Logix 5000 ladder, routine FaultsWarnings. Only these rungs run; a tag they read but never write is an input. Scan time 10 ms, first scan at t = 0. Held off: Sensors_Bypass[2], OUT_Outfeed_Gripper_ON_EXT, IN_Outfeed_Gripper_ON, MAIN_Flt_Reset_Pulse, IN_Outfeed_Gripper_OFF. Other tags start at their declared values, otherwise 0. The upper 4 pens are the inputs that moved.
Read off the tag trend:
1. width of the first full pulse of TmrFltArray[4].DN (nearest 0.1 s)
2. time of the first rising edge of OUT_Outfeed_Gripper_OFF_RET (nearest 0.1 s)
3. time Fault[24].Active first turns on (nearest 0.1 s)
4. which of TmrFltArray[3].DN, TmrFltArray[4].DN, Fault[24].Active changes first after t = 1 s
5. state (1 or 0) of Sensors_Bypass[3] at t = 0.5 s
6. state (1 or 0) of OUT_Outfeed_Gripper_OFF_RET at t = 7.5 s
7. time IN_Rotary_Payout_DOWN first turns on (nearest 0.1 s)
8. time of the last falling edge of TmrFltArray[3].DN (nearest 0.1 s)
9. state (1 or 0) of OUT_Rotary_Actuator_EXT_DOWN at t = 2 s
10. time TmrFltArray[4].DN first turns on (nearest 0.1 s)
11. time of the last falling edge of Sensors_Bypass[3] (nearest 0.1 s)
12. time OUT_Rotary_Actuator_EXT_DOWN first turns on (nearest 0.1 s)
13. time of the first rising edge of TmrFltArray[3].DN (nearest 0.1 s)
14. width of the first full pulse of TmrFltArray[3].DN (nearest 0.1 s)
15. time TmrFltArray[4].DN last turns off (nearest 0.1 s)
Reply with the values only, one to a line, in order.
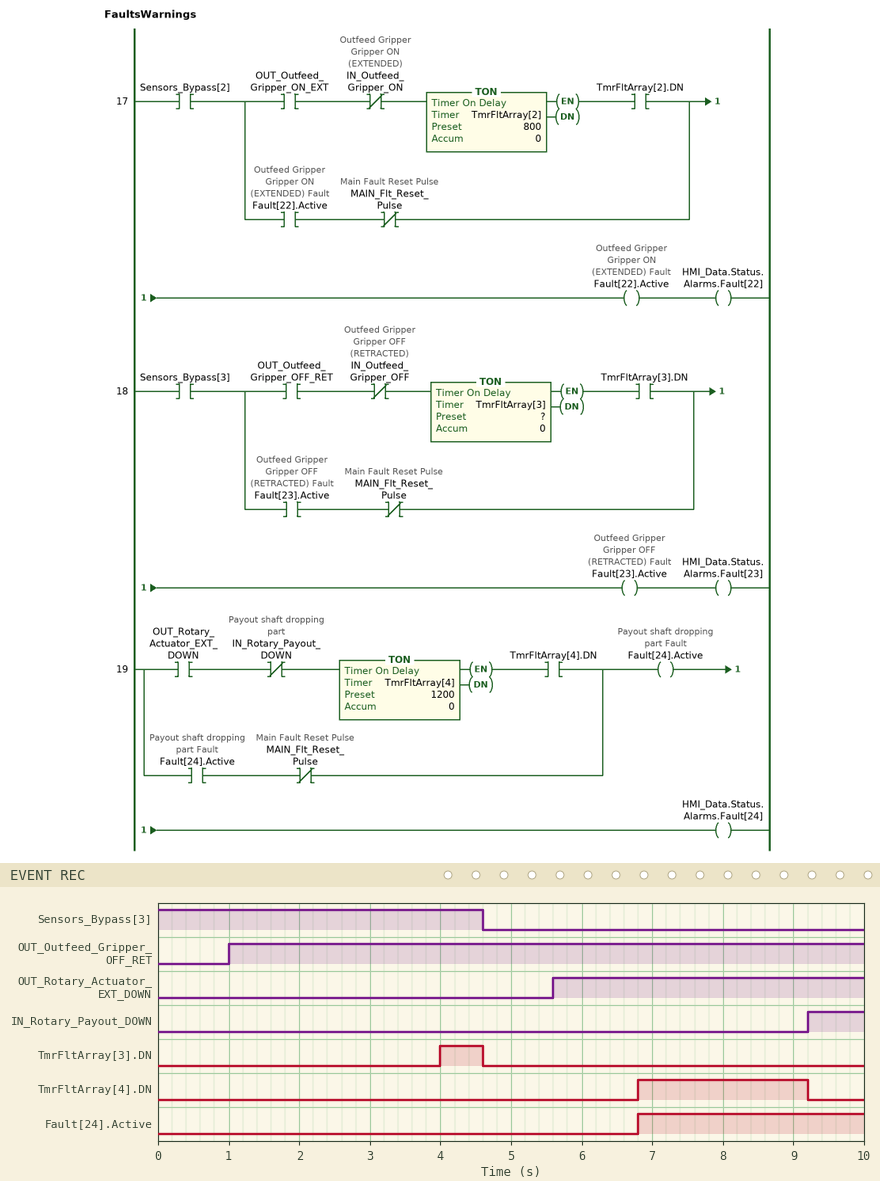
2.4 s
1.0 s
6.8 s
TmrFltArray[3].DN
1
1
9.2 s
4.6 s
0
6.8 s
4.6 s
5.6 s
4.0 s
0.6 s
9.2 s
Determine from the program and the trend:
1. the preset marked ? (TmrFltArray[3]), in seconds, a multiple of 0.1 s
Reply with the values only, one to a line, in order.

3.0 s
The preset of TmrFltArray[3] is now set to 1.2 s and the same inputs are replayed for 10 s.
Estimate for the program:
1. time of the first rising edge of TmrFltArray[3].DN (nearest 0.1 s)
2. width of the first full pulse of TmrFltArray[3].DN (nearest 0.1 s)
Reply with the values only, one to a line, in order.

2.2 s
2.4 s
